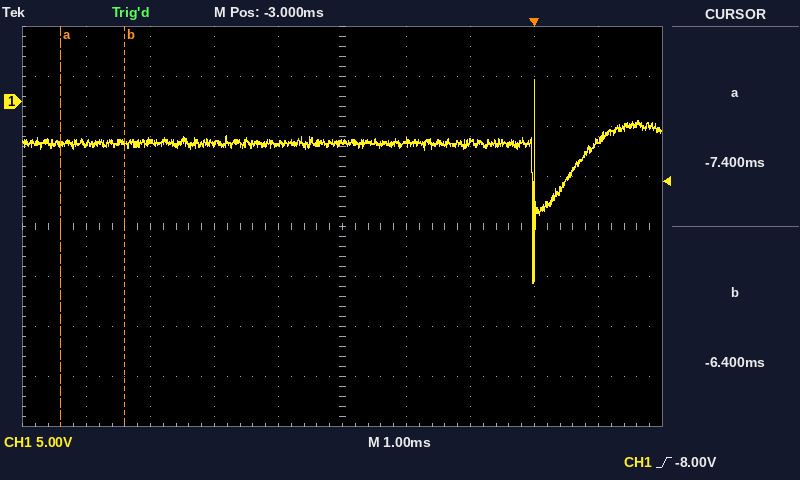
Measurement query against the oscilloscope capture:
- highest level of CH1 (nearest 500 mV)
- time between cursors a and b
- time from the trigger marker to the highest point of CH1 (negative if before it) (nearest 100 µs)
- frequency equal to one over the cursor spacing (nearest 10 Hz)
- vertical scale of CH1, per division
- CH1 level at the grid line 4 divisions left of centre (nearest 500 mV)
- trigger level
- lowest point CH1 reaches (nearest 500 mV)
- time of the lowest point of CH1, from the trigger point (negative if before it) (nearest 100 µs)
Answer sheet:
2.0 V
1.0 ms
0.0 ms
1.00 kHz
5 V
-4.0 V
-8.00 V
-18.0 V
0.0 ms
